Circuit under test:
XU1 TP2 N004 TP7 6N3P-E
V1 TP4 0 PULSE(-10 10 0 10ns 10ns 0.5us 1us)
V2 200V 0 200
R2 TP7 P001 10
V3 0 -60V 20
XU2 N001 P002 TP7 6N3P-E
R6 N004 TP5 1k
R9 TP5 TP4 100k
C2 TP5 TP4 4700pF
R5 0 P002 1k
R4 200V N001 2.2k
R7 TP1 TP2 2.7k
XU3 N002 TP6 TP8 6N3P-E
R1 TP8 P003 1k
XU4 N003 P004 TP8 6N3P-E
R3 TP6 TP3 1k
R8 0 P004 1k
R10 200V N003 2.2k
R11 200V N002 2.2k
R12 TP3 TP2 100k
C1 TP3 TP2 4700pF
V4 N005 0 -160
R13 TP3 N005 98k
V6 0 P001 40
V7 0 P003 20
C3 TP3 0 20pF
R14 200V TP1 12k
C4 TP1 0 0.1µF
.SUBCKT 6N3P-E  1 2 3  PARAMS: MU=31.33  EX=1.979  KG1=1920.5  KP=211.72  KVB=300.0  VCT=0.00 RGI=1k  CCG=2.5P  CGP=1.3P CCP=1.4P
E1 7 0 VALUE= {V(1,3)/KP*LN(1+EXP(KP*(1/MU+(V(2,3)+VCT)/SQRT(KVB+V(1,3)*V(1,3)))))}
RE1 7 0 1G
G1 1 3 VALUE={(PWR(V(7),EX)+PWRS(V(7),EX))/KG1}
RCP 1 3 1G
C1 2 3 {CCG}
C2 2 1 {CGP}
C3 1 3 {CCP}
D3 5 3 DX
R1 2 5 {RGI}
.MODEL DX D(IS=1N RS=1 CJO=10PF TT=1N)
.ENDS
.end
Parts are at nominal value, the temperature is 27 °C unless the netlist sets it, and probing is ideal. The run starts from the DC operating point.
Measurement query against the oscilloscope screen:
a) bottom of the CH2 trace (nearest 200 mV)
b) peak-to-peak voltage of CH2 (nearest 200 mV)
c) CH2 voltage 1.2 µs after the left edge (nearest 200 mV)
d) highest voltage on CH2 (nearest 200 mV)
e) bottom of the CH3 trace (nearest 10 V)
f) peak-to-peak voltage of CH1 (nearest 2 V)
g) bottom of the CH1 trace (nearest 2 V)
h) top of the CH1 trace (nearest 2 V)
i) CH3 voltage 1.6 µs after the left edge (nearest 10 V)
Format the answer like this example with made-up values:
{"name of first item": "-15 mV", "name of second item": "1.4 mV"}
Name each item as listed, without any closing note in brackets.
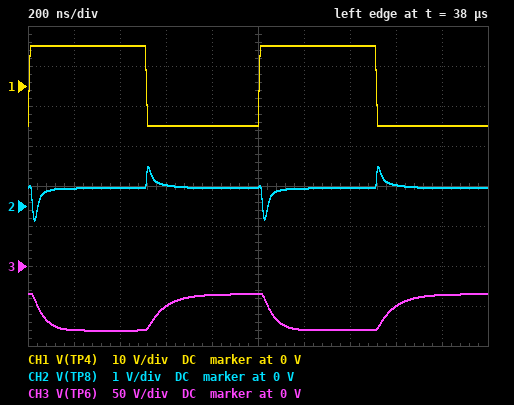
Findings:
{"bottom of the CH2 trace": "-400 mV", "peak-to-peak voltage of CH2": "1.4 V", "CH2 voltage 1.2 µs after the left edge": "400 mV", "highest voltage on CH2": "1.0 V", "bottom of the CH3 trace": "-80 V", "peak-to-peak voltage of CH1": "20 V", "bottom of the CH1 trace": "-10 V", "top of the CH1 trace": "10 V", "CH3 voltage 1.6 µs after the left edge": "-50 V"}
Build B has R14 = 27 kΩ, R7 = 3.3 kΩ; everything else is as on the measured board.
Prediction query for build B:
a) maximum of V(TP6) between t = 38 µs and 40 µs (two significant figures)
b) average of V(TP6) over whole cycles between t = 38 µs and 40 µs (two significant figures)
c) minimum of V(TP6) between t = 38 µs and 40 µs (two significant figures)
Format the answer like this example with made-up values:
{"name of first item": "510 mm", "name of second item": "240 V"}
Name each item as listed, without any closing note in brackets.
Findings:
{"maximum of V(TP6) between t = 38 µs and 40 µs": "-57 V", "average of V(TP6) over whole cycles between t = 38 µs and 40 µs": "-73 V", "minimum of V(TP6) between t = 38 µs and 40 µs": "-86 V"}
